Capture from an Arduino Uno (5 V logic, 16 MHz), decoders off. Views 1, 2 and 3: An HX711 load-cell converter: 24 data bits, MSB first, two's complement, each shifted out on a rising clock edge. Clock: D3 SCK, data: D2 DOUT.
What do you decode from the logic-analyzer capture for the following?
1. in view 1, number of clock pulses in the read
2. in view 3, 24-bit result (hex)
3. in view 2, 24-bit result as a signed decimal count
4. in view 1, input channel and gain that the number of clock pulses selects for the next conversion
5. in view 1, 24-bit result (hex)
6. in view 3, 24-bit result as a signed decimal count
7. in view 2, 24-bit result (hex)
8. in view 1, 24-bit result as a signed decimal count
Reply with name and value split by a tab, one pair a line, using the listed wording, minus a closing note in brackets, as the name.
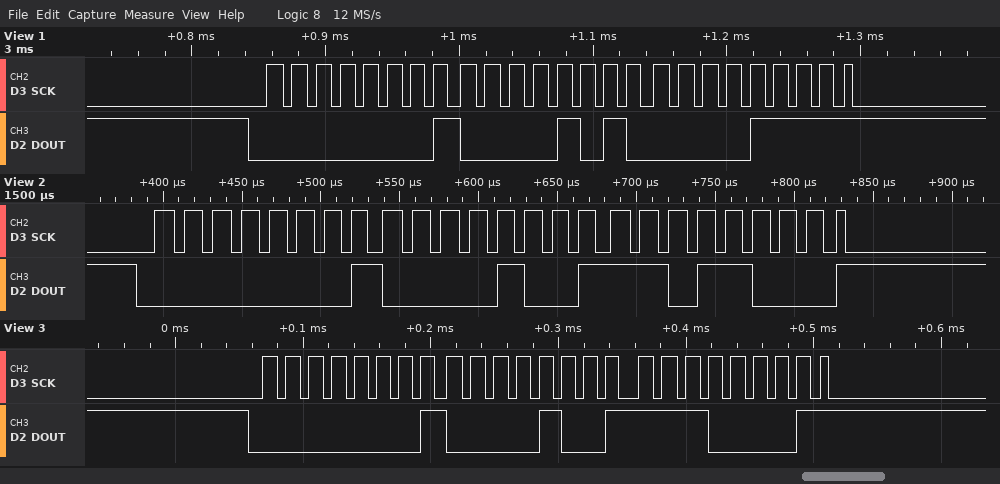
in view 1, number of clock pulses in the read	25
in view 3, 24-bit result	0x0109E1
in view 2, 24-bit result as a signed decimal count	68056
in view 1, input channel and gain that the number of clock pulses selects for the next conversion	channel A, gain 128
in view 1, 24-bit result	0x010A0F
in view 3, 24-bit result as a signed decimal count	68065
in view 2, 24-bit result	0x0109D8
in view 1, 24-bit result as a signed decimal count	68111
